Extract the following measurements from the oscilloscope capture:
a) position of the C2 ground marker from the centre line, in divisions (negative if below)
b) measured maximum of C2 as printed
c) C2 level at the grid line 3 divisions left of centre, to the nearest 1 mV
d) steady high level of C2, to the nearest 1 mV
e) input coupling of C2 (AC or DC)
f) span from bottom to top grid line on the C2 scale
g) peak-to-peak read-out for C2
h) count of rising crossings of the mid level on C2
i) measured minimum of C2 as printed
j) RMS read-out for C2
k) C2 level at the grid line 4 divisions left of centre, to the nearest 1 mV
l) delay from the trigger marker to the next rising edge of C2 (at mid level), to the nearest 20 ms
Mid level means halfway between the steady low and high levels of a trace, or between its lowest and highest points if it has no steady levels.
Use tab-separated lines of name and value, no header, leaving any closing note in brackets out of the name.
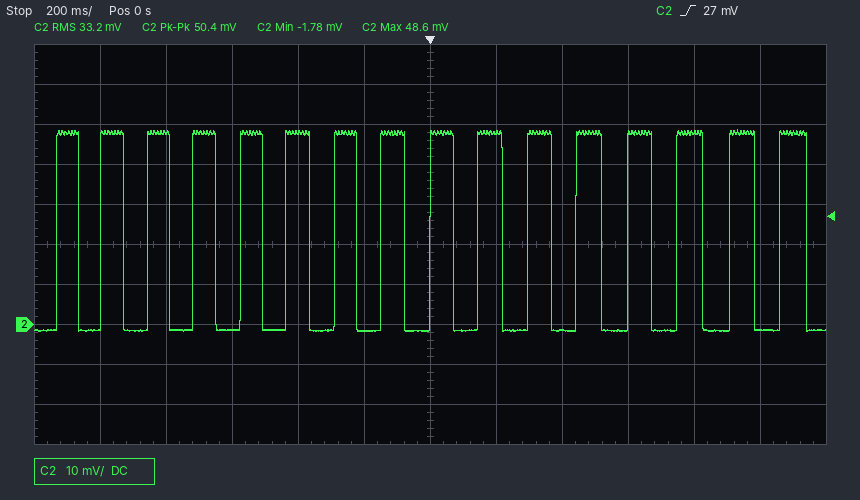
position of the C2 ground marker from the centre line, in divisions	-2.0 div
measured maximum of C2 as printed	48.6 mV
C2 level at the grid line 3 divisions left of centre, to the nearest 1 mV	-1 mV
steady high level of C2, to the nearest 1 mV	48 mV
input coupling of C2	DC
span from bottom to top grid line on the C2 scale	100 mV
peak-to-peak read-out for C2	50.4 mV
count of rising crossings of the mid level on C2	16
measured minimum of C2 as printed	-1.78 mV
RMS read-out for C2	33.2 mV
C2 level at the grid line 4 divisions left of centre, to the nearest 1 mV	48 mV
delay from the trigger marker to the next rising edge of C2 (at mid level), to the nearest 20 ms	140 ms
